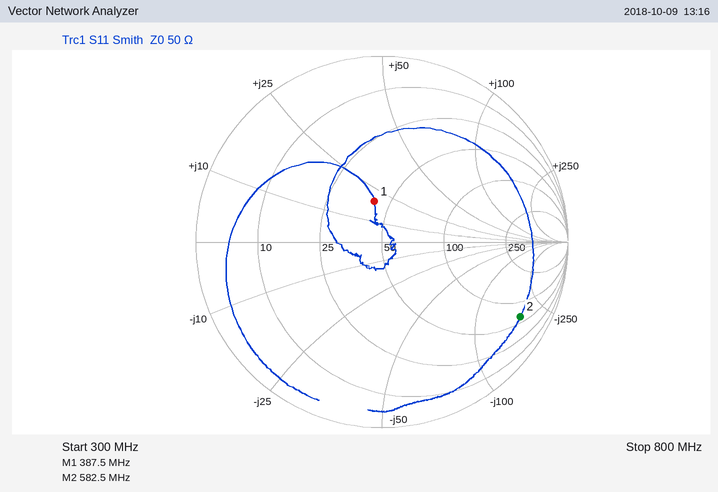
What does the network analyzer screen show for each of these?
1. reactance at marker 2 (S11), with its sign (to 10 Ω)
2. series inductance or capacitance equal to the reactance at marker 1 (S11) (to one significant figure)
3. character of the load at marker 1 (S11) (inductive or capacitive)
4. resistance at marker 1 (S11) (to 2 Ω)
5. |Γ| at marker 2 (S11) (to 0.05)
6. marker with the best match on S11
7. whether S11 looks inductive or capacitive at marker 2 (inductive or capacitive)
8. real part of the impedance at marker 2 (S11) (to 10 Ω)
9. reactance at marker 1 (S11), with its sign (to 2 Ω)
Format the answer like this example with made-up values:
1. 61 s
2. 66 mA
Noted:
1. -180 Ω
2. 8 nH
3. inductive
4. 42 Ω
5. 0.85
6. marker 1
7. capacitive
8. 60 Ω
9. +20 Ω
